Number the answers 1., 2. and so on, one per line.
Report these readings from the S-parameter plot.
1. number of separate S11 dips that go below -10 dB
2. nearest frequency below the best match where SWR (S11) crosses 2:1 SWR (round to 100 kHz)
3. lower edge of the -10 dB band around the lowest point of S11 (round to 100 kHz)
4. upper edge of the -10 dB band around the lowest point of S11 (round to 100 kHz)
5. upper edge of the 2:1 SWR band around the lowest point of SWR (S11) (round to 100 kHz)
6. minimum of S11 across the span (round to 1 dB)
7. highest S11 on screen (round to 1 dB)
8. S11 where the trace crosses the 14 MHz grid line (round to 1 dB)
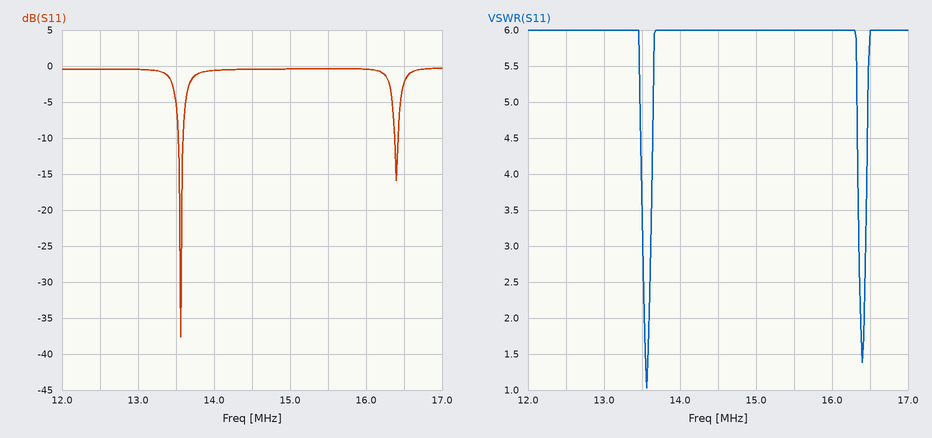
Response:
1. 2
2. 13.5 MHz
3. 13.5 MHz
4. 13.6 MHz
5. 13.6 MHz
6. -38 dB
7. 0 dB
8. -1 dB
